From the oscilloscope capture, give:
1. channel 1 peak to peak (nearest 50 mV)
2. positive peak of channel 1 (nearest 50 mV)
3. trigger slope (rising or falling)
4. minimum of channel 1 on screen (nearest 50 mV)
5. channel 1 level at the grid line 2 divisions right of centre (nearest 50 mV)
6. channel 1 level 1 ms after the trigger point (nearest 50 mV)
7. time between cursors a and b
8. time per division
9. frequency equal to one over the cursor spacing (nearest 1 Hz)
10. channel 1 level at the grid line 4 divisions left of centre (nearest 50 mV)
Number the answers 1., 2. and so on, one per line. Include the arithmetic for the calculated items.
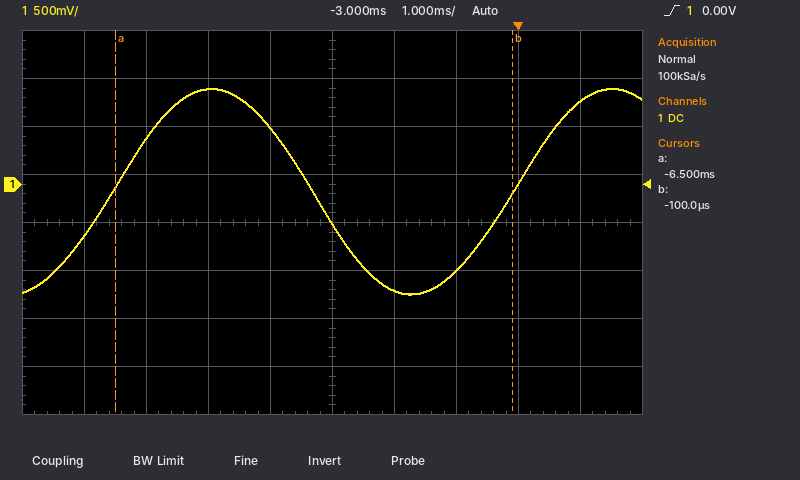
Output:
1. 1.00 V − (-1.15 V) = 2.15 V
2. 1.00 V
3. rising
4. -1.15 V
5. -900 mV
6. 850 mV
7. -100 µs − (-6.5 ms) = 6.4 ms
8. 1 ms
9. 1 / 6.4 ms ≈ 156 Hz
10. -550 mV
